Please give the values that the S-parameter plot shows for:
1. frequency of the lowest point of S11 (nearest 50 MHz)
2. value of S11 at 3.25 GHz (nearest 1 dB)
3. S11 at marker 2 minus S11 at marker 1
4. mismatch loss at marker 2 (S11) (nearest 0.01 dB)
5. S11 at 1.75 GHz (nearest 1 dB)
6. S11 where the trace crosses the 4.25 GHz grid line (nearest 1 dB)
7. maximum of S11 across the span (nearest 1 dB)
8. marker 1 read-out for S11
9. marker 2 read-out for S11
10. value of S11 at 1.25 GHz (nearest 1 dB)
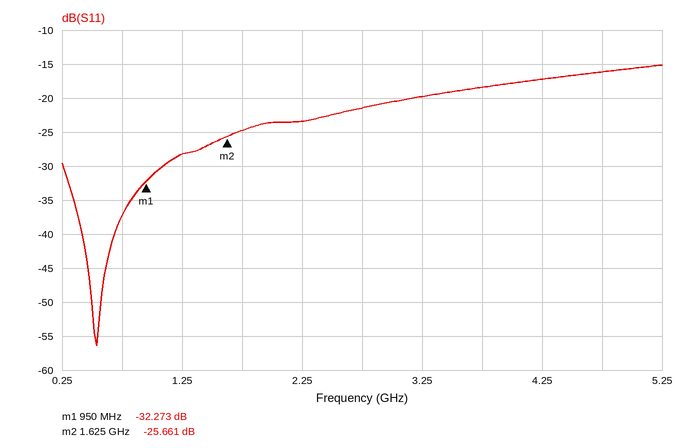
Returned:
550 MHz
-20 dB
6.612 dB
0.01 dB
-25 dB
-17 dB
-15 dB
-32.273 dB
-25.661 dB
-28 dB
